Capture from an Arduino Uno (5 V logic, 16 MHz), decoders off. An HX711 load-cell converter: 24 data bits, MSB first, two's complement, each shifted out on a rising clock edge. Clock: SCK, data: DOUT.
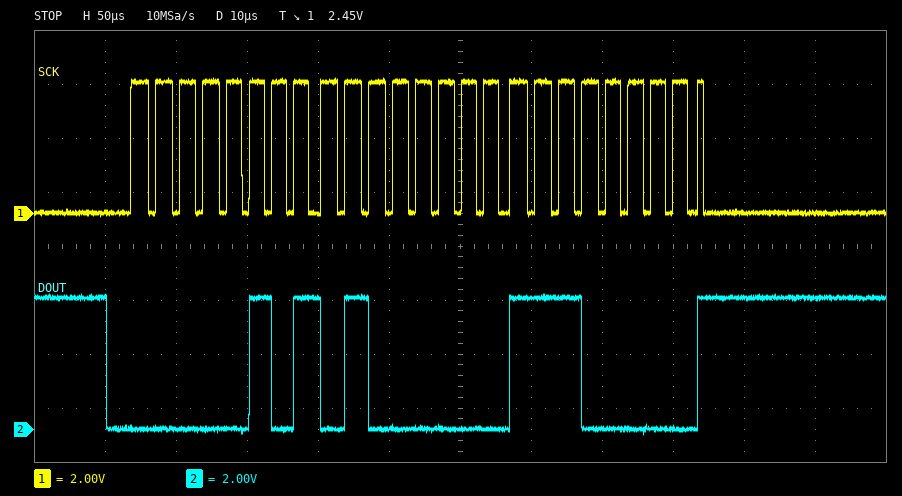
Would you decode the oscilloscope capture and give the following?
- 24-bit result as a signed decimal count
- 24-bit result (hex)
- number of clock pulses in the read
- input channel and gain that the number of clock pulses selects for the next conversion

344288
0x0540E0
25
channel A, gain 128
